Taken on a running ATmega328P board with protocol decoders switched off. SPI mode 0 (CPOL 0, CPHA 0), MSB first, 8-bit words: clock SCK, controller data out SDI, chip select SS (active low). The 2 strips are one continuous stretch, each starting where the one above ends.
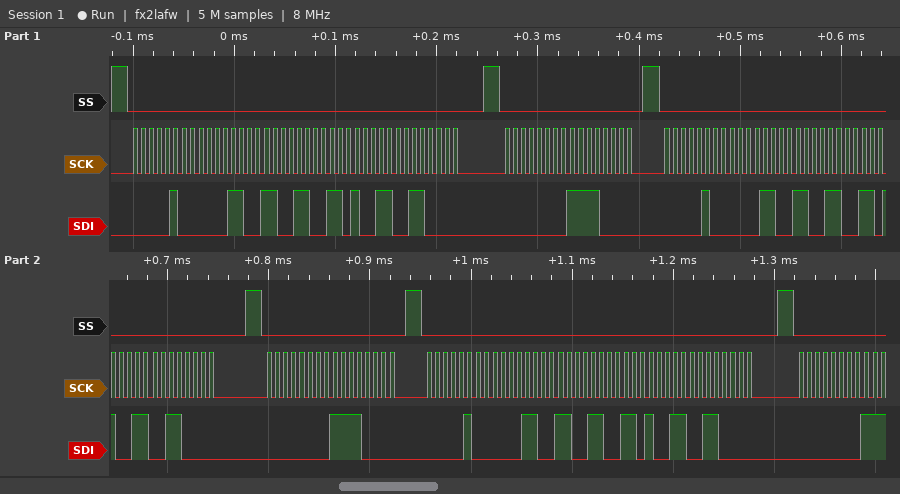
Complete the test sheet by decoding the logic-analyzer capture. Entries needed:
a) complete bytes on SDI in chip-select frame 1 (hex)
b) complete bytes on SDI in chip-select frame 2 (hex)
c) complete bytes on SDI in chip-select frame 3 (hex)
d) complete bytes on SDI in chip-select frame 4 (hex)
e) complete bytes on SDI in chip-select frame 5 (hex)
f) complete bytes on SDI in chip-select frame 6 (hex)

04 0C CC D3 30
00 F0
04 0C CC D3 30
00 F0
04 0C CC D3 30
00
